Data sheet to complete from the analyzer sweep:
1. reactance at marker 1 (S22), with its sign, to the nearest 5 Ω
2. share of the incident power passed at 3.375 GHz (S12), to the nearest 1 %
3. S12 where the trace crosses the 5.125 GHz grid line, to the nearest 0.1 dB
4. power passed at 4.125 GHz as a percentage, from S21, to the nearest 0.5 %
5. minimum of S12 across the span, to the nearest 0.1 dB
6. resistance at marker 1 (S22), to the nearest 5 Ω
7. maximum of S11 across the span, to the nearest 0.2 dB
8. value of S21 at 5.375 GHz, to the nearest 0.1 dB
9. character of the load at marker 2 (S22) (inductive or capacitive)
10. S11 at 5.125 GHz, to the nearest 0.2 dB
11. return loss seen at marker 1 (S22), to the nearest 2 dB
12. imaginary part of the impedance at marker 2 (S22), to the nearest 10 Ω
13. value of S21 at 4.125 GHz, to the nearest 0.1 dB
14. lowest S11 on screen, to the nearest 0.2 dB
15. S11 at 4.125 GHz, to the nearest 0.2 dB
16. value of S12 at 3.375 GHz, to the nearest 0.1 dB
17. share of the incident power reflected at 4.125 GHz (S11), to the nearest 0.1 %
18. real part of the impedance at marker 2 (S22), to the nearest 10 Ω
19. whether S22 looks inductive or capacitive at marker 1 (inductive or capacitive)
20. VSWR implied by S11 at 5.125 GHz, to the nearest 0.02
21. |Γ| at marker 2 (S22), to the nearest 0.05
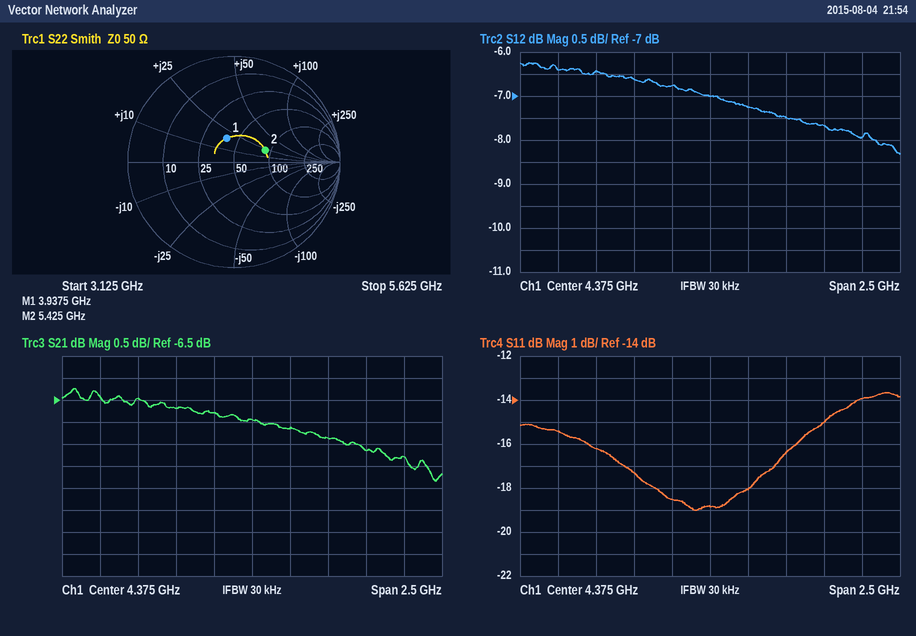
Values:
+20 Ω
23 %
-7.7 dB
21.0 %
-8.3 dB
40 Ω
-13.6 dB
-7.8 dB
inductive
-15.0 dB
12 dB
+20 Ω
-6.8 dB
-19.0 dB
-18.6 dB
-6.4 dB
1.4 %
90 Ω
inductive
1.44
0.30
